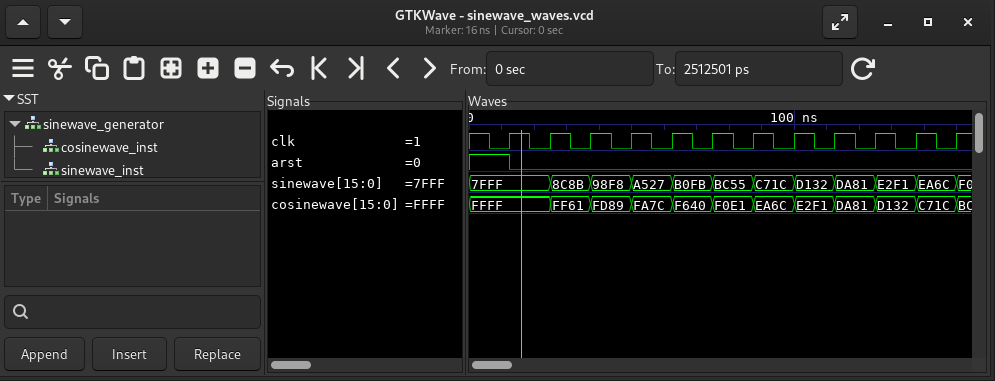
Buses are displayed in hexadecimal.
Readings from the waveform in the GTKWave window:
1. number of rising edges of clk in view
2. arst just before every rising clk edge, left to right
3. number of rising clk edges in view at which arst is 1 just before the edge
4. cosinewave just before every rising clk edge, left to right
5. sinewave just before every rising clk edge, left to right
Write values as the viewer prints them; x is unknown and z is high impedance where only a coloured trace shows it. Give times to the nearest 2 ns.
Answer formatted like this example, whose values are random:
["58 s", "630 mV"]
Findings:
["12", "1 0 0 0 0 0 0 0 0 0 0 0", "1", "FFFF, FFFF, FF61, FD89, FA7C, F640, F0E1, EA6C, E2F1, DA81, D132, C71C", "7FFF, 7FFF, 8C8B, 98F8, A527, B0FB, BC55, C71C, D132, DA81, E2F1, EA6C"]
